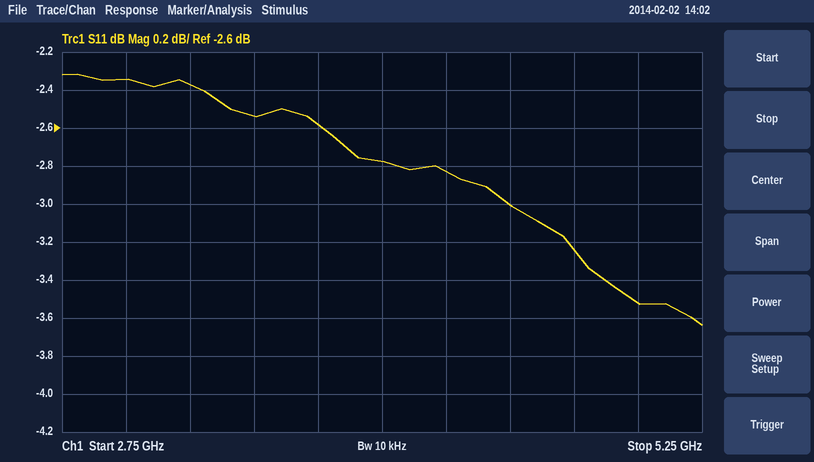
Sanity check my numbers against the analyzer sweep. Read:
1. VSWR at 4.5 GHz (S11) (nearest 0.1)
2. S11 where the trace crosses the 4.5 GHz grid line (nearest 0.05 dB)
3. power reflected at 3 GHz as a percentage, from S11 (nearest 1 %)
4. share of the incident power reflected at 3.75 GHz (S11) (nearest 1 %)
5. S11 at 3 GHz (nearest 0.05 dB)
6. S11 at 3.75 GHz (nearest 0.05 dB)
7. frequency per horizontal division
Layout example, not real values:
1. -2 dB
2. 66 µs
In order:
1. 5.8
2. -3.00 dB
3. 58 %
4. 55 %
5. -2.35 dB
6. -2.60 dB
7. 250 MHz
